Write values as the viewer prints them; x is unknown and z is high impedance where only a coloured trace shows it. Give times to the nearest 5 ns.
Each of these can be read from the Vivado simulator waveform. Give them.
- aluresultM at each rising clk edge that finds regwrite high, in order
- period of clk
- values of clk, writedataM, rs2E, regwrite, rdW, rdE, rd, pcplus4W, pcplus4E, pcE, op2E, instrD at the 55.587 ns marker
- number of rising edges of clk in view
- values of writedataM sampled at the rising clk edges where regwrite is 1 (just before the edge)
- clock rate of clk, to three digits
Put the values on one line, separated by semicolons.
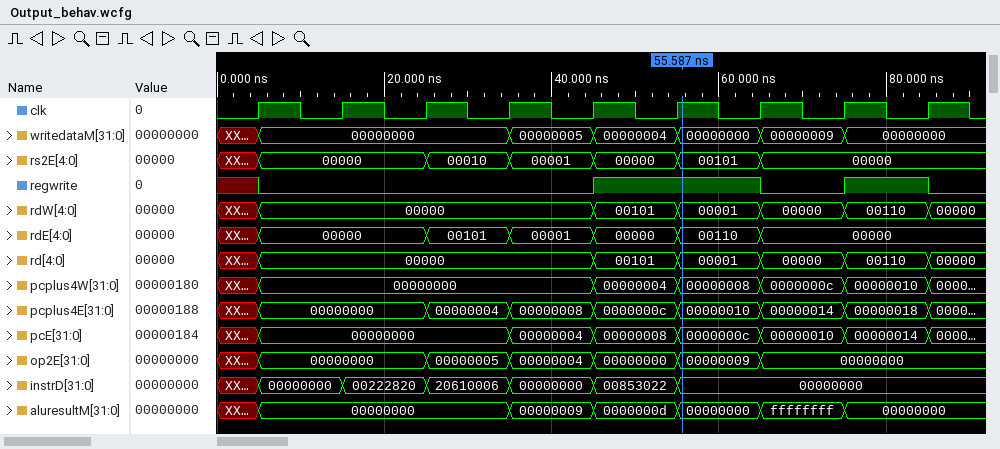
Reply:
0000000d, 00000000, 00000000; 10 ns; clk=1, writedataM=00000000, rs2E=00101, regwrite=1, rdW=00001, rdE=00110, rd=00001, pcplus4W=00000008, pcplus4E=00000010, pcE=0000000c, op2E=00000009, instrD=00000000; 9; 00000004, 00000000, 00000000; 100 MHz
